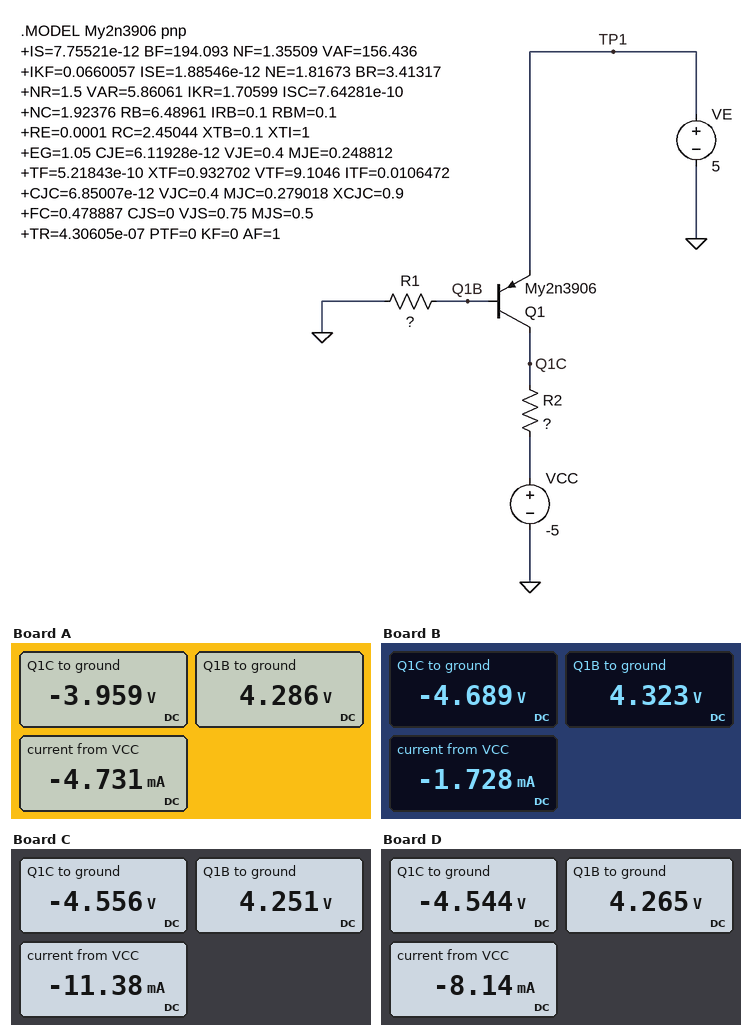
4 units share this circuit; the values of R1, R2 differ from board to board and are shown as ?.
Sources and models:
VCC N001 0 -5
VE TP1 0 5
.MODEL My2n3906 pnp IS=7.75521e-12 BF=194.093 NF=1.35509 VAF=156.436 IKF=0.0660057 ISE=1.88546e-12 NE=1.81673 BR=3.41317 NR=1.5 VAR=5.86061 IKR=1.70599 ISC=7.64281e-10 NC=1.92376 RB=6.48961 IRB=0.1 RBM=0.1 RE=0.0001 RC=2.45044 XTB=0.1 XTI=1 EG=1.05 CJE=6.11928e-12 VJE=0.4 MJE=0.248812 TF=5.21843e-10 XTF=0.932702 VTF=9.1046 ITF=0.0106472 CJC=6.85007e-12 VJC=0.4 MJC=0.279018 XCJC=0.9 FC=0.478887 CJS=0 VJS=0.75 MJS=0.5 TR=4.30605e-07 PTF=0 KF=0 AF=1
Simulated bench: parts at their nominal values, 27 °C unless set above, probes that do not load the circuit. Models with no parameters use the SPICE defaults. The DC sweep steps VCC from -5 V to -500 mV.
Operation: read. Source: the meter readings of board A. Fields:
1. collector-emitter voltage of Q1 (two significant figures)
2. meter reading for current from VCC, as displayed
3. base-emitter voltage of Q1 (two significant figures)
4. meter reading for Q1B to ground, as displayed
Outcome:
-9.0 V
-4.731 mA
-710 mV
4.286 V
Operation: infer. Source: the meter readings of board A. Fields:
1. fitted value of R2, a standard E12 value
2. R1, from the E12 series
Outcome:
220 Ω
120 kΩ
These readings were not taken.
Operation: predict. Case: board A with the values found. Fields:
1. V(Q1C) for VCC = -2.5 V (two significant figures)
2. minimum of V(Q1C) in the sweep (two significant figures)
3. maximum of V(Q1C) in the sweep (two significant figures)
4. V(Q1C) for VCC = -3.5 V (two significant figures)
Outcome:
-1.5 V
-4.0 V
510 mV
-2.5 V
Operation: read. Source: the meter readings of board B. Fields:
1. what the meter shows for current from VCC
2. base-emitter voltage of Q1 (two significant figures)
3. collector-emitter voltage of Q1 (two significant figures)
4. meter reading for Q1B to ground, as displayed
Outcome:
-1.728 mA
-680 mV
-9.7 V
4.323 V
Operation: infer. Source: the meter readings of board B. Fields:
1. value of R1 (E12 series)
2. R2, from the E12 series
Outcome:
330 kΩ
180 Ω
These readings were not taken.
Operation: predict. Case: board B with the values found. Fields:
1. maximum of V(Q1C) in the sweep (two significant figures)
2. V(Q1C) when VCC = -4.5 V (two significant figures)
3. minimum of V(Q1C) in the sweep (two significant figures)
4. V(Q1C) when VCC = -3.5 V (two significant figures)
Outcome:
-200 mV
-4.2 V
-4.7 V
-3.2 V
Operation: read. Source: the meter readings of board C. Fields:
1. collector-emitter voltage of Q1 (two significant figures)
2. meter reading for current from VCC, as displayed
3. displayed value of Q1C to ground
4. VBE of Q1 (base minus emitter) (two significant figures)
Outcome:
-9.6 V
-11.38 mA
-4.556 V
-750 mV
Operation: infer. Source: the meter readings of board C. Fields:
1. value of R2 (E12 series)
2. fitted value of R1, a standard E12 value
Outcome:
39 Ω
47 kΩ
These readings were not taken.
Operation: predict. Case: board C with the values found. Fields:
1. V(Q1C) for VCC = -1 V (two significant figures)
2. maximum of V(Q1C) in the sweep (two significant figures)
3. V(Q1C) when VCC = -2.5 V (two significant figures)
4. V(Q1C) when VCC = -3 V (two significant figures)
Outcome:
-570 mV
-70 mV
-2.1 V
-2.6 V
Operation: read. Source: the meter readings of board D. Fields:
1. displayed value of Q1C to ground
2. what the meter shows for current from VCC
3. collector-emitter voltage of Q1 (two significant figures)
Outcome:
-4.544 V
-8.14 mA
-9.5 V
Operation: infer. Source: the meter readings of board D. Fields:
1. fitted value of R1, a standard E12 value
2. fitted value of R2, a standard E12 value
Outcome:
68 kΩ
56 Ω
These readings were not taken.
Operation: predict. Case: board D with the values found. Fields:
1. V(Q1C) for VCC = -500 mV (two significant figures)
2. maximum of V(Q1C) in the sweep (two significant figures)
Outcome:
-58 mV
-58 mV
